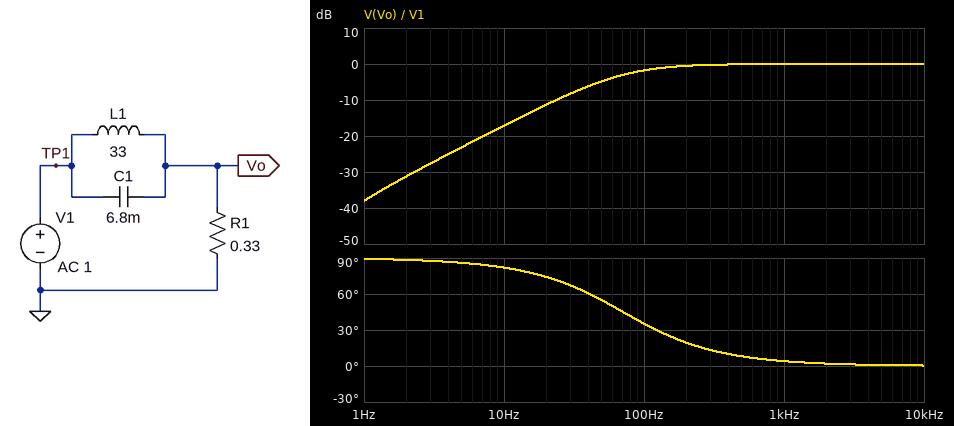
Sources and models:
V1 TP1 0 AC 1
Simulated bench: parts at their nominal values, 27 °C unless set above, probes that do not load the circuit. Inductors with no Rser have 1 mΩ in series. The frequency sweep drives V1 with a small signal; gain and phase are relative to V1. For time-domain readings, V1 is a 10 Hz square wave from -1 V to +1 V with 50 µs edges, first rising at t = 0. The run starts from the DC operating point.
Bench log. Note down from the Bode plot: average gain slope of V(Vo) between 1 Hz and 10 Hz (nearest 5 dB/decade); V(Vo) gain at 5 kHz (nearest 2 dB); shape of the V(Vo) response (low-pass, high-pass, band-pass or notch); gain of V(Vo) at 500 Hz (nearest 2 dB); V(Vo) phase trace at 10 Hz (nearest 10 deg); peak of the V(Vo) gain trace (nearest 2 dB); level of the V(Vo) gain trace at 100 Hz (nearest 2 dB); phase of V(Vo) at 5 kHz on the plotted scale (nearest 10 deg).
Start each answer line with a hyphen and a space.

- 20 dB/decade
- 0 dB
- high-pass
- 0 dB
- 80 deg
- 0 dB
- -2 dB
- 0 deg
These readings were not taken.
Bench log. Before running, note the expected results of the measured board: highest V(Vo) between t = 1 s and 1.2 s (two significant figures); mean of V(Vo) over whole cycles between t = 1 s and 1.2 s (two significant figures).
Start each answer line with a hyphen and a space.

- 990 mV
- -990 mV
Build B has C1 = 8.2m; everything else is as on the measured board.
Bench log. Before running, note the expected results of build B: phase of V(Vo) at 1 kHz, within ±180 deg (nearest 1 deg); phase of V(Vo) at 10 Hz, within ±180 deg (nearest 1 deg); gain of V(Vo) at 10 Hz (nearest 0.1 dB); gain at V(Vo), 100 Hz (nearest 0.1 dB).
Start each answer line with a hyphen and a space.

- 3 deg
- 80 deg
- -15.5 dB
- -1.3 dB
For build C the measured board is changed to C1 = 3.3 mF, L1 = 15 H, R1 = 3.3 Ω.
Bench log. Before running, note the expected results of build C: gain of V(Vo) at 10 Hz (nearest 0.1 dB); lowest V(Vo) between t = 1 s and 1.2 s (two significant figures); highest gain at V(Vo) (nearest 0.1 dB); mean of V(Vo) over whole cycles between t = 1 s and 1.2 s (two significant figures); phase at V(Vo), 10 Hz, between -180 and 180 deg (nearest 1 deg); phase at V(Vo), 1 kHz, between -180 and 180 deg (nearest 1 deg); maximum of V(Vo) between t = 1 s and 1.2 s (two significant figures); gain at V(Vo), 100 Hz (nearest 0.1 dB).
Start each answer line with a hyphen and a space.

- -5.0 dB
- -2.8 V
- 0 dB
- -780 mV
- 56 deg
- 1 deg
- 1.2 V
- -0.1 dB
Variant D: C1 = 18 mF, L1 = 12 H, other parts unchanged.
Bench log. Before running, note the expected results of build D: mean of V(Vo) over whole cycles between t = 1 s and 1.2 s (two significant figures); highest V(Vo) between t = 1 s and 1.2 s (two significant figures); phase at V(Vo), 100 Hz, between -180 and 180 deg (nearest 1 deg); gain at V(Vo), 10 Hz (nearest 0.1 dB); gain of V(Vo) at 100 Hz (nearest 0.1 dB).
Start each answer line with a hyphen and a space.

- -970 mV
- 1.0 V
- 15 deg
- -9.1 dB
- -0.3 dB
